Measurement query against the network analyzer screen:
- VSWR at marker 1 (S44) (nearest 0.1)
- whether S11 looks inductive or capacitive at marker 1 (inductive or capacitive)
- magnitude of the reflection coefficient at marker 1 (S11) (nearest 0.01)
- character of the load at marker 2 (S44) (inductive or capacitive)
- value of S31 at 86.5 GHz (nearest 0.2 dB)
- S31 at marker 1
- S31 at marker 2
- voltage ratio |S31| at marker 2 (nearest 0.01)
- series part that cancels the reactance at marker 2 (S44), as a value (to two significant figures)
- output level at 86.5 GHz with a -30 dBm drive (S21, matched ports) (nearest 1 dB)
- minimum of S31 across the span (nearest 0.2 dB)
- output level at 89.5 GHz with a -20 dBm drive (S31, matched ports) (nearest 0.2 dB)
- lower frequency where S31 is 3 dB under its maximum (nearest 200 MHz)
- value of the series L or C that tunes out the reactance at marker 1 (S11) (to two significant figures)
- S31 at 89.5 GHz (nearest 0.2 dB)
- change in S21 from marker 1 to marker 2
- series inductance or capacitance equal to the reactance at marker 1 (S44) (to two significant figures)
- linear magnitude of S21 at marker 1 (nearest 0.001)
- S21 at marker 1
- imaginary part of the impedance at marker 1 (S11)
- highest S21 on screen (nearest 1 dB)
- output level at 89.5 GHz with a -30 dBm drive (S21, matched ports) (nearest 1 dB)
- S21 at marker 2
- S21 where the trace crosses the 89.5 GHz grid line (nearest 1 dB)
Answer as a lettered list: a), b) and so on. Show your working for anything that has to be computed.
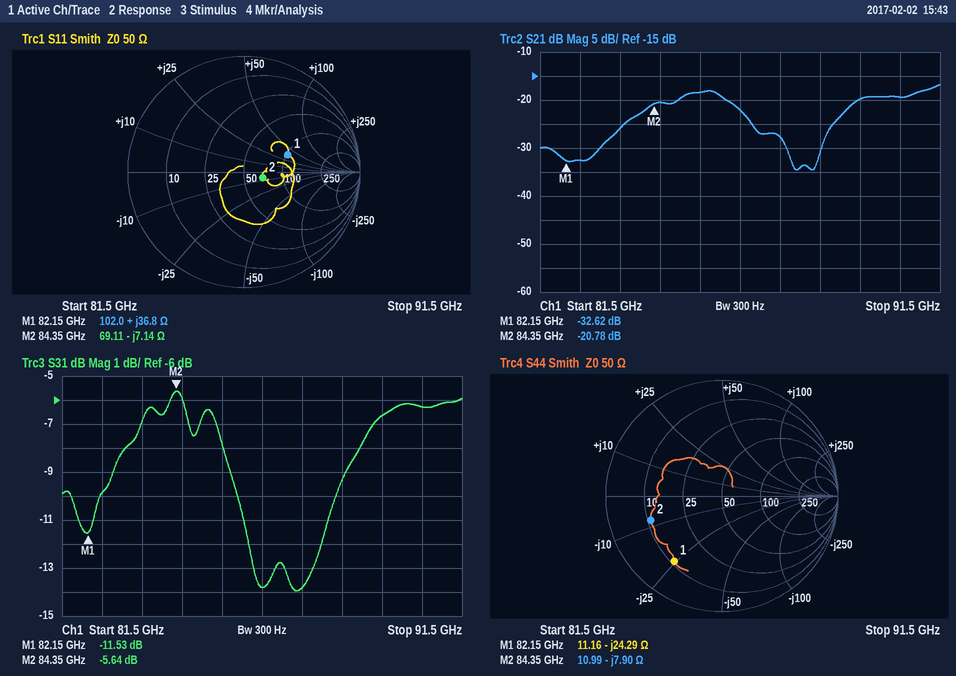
a) 5.6
b) inductive
c) 0.41
d) capacitive
e) -13.8 dB
f) -11.53 dB
g) -5.64 dB
h) 10^(-5.64/20) ≈ 0.52
i) L = 7.9 Ω/(2π × 84.35 GHz) ≈ 15 pH
j) -30 dBm + (-22 dB) = -52 dBm
k) -14.0 dB
l) -20 dBm + (-6.6 dB) = -26.6 dBm
m) 82.8 GHz
n) C = 1/(2π × 82.15 GHz × 36.8 Ω) ≈ 53 fF
o) -6.6 dB
p) -20.78 − (-32.62) = 11.84 dB
q) C = 1/(2π × 82.15 GHz × 24.29 Ω) ≈ 80 fF
r) 10^(-32.62/20) ≈ 0.023
s) -32.62 dB
t) +36.8 Ω
u) -17 dB
v) -30 dBm + (-20 dB) = -50 dBm
w) -20.78 dB
x) -20 dB
